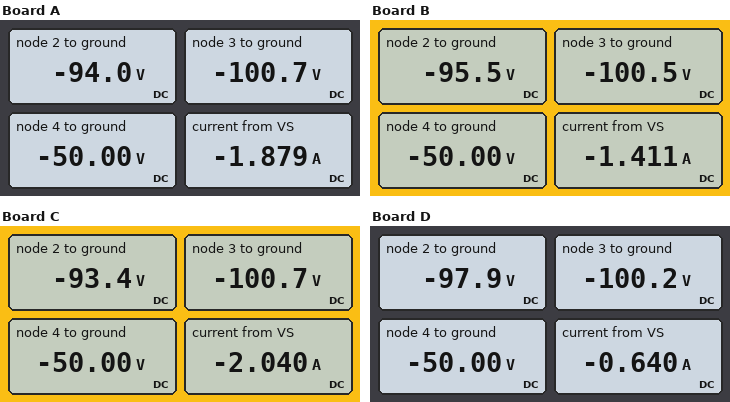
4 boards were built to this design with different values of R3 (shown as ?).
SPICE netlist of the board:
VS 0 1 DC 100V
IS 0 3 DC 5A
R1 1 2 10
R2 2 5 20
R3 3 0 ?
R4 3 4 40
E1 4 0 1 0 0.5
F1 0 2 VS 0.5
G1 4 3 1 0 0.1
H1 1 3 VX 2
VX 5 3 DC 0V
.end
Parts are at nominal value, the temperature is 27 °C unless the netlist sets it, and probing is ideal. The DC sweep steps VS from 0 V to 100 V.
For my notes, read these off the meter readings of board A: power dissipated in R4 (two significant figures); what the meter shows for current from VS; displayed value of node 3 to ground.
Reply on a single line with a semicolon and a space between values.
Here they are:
64 W; -1.879 A; -100.7 V
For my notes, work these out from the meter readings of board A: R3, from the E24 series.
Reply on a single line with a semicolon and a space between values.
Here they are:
110 Ω
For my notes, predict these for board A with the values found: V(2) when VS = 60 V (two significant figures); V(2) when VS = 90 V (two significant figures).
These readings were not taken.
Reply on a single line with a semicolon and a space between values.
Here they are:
-61 V; -86 V
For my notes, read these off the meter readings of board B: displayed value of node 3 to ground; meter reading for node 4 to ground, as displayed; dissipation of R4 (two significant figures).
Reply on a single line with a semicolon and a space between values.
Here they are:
-100.5 V; -50.00 V; 64 W
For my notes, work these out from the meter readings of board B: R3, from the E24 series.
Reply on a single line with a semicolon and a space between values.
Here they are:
62 Ω
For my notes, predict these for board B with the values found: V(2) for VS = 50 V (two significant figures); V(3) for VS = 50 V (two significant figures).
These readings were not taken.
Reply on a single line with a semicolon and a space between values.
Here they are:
-53 V; -50 V
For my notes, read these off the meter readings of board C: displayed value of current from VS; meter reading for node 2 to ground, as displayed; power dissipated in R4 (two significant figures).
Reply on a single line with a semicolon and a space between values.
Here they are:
-2.040 A; -93.4 V; 64 W
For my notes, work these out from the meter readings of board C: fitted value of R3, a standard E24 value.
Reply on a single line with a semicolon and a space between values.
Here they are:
150 Ω
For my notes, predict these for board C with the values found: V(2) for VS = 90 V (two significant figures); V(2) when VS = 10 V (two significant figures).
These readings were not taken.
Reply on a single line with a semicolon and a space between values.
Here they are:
-85 V; -19 V
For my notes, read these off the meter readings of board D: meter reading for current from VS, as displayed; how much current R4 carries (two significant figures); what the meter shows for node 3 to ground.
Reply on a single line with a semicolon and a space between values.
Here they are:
-0.640 A; 1.3 A; -100.2 V
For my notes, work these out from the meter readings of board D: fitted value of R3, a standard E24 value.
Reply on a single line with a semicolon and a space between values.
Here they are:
36 Ω
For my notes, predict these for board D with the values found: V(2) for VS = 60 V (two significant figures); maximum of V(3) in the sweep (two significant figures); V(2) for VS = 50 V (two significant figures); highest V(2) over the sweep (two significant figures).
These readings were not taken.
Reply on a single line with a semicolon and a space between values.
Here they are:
-63 V; 1.2 V; -54 V; -11 V
